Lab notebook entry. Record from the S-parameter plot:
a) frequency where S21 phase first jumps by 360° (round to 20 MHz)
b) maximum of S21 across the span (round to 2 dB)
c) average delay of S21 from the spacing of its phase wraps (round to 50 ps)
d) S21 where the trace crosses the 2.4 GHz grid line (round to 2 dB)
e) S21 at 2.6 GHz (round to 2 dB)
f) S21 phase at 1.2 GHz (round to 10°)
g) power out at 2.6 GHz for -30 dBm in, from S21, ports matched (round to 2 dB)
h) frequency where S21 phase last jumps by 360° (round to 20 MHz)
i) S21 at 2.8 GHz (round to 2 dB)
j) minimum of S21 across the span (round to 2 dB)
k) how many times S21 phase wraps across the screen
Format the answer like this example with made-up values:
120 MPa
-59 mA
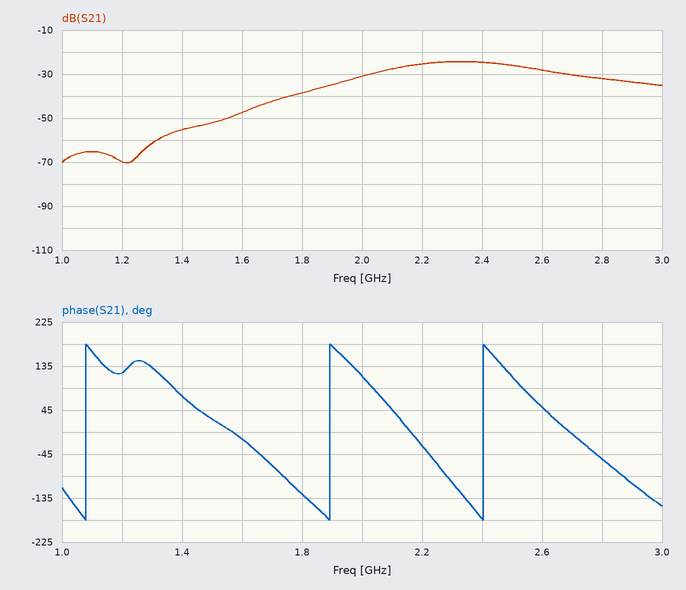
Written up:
1.08 GHz
-24 dB
1.50 ns
-24 dB
-28 dB
120°
-58 dBm
2.40 GHz
-32 dB
-70 dB
3
